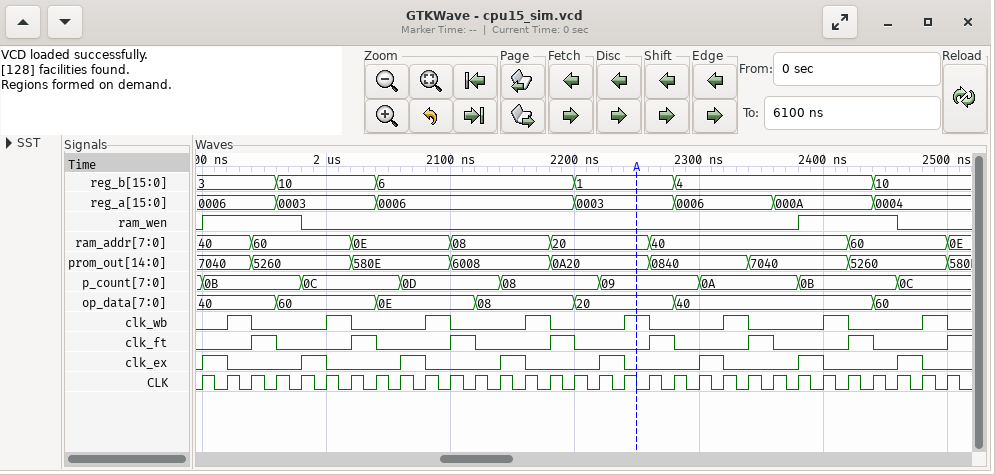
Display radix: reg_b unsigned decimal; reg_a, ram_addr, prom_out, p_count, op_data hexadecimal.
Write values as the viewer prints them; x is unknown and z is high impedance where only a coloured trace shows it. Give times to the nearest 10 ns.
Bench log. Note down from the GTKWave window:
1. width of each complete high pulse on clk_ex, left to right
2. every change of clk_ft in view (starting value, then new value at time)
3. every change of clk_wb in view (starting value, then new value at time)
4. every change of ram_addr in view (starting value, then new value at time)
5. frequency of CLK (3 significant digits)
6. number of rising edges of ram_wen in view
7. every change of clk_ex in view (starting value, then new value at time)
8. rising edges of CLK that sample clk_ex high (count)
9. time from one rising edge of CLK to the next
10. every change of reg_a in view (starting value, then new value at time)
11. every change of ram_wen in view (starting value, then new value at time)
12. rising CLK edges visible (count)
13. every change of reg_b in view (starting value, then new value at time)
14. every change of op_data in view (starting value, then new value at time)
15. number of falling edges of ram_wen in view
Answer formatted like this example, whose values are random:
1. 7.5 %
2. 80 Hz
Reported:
1. 20 ns, 20 ns, 20 ns, 20 ns, 20 ns, 20 ns, 20 ns, 20 ns
2. 0, 1 at 1940 ns, 0 at 1960 ns, 1 at 2020 ns, 0 at 2040 ns, 1 at 2100 ns, 0 at 2120 ns, 1 at 2180 ns, 0 at 2200 ns, 1 at 2260 ns, 0 at 2280 ns, 1 at 2340 ns, 0 at 2360 ns, 1 at 2420 ns, 0 at 2440 ns, 1 at 2500 ns
3. 0, 1 at 1920 ns, 0 at 1940 ns, 1 at 2000 ns, 0 at 2020 ns, 1 at 2080 ns, 0 at 2100 ns, 1 at 2160 ns, 0 at 2180 ns, 1 at 2240 ns, 0 at 2260 ns, 1 at 2320 ns, 0 at 2340 ns, 1 at 2400 ns, 0 at 2420 ns, 1 at 2480 ns, 0 at 2500 ns
4. 40, 60 at 1940 ns, 0E at 2020 ns, 08 at 2100 ns, 20 at 2180 ns, 40 at 2260 ns, 60 at 2420 ns, 0E at 2500 ns
5. 50.0 MHz
6. 2
7. 0, 1 at 1900 ns, 0 at 1920 ns, 1 at 1980 ns, 0 at 2000 ns, 1 at 2060 ns, 0 at 2080 ns, 1 at 2140 ns, 0 at 2160 ns, 1 at 2220 ns, 0 at 2240 ns, 1 at 2300 ns, 0 at 2320 ns, 1 at 2380 ns, 0 at 2400 ns, 1 at 2460 ns, 0 at 2480 ns
8. 8
9. 20 ns
10. 0006, 0003 at 1960 ns, 0006 at 2040 ns, 0003 at 2200 ns, 0006 at 2280 ns, 000A at 2360 ns, 0004 at 2440 ns
11. 0, 1 at 1900 ns, 0 at 1980 ns, 1 at 2380 ns, 0 at 2460 ns
12. 31
13. 3, 10 at 1960 ns, 6 at 2040 ns, 1 at 2200 ns, 4 at 2280 ns, 10 at 2440 ns
14. 40, 60 at 1960 ns, 0E at 2040 ns, 08 at 2120 ns, 20 at 2200 ns, 40 at 2280 ns, 60 at 2440 ns
15. 2
